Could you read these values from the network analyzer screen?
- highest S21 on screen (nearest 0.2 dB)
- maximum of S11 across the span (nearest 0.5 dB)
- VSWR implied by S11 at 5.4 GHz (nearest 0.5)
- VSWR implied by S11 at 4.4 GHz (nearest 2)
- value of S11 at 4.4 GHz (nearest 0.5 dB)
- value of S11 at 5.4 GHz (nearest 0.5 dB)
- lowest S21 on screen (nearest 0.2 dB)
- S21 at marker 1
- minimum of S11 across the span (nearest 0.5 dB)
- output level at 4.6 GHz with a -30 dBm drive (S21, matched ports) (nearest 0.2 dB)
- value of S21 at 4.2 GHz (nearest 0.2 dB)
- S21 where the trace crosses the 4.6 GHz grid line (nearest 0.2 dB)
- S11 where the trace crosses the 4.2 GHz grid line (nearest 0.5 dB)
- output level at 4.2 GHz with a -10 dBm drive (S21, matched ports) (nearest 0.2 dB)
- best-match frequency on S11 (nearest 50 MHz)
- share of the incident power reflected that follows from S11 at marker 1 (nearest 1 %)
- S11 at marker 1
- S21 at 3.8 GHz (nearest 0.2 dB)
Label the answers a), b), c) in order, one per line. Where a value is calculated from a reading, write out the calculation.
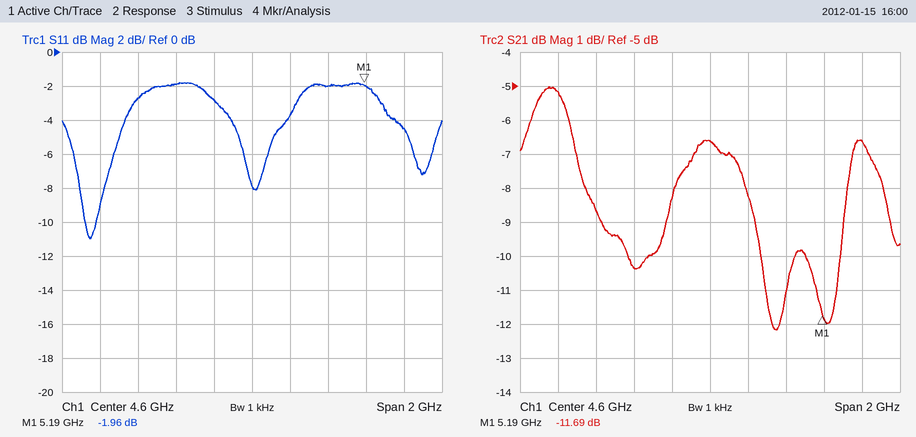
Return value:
a) -5.0 dB
b) -2.0 dB
c) |Γ| = 10^(-4.5/20) = 0.5957; VSWR = (1 + 0.5957)/(1 − 0.5957) ≈ 4.0
d) |Γ| = 10^(-3/20) = 0.7079; VSWR = (1 + 0.7079)/(1 − 0.7079) ≈ 6
e) -3.0 dB
f) -4.5 dB
g) -12.2 dB
h) -11.69 dB
i) -11.0 dB
j) -30 dBm + (-6.6 dB) = -36.6 dBm
k) -10.4 dB
l) -6.6 dB
m) -2.0 dB
n) -10 dBm + (-10.4 dB) = -20.4 dBm
o) 3.75 GHz
p) 10^(-1.96/10) ≈ 64 %
q) -1.96 dB
r) -5.2 dB
